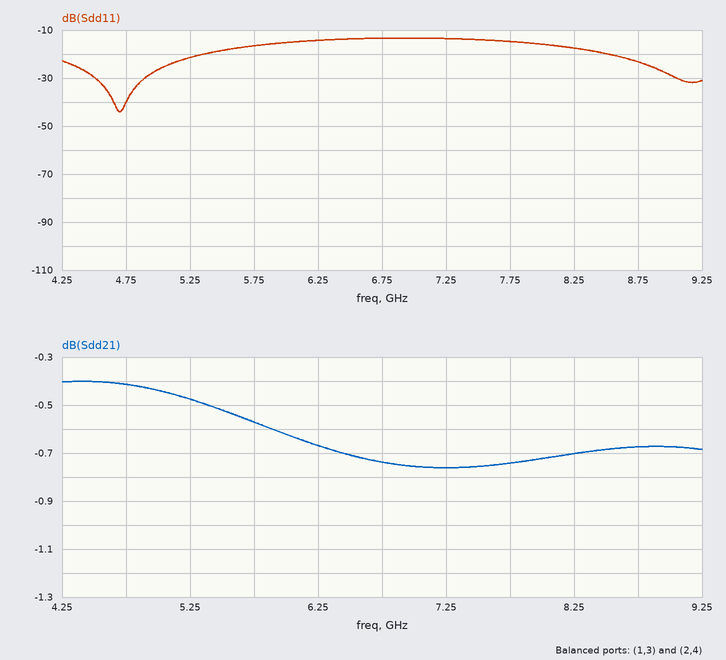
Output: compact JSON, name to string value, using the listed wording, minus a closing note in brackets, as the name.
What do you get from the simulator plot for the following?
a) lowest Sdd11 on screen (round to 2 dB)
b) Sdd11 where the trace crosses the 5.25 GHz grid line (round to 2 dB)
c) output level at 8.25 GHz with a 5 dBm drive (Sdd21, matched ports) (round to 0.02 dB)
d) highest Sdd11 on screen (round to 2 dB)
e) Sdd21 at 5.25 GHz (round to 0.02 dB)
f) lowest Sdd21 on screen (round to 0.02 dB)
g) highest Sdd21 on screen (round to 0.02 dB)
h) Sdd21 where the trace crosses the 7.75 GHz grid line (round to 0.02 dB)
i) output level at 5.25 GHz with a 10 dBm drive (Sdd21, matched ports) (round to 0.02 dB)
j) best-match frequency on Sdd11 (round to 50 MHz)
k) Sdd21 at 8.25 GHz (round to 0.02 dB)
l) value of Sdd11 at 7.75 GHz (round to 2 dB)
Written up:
{"lowest Sdd11 on screen": "-44 dB", "Sdd11 where the trace crosses the 5.25 GHz grid line": "-22 dB", "output level at 8.25 GHz with a 5 dBm drive (Sdd21, matched ports)": "4.30 dBm", "highest Sdd11 on screen": "-14 dB", "Sdd21 at 5.25 GHz": "-0.48 dB", "lowest Sdd21 on screen": "-0.76 dB", "highest Sdd21 on screen": "-0.40 dB", "Sdd21 where the trace crosses the 7.75 GHz grid line": "-0.74 dB", "output level at 5.25 GHz with a 10 dBm drive (Sdd21, matched ports)": "9.52 dBm", "best-match frequency on Sdd11": "4.70 GHz", "Sdd21 at 8.25 GHz": "-0.70 dB", "value of Sdd11 at 7.75 GHz": "-14 dB"}
